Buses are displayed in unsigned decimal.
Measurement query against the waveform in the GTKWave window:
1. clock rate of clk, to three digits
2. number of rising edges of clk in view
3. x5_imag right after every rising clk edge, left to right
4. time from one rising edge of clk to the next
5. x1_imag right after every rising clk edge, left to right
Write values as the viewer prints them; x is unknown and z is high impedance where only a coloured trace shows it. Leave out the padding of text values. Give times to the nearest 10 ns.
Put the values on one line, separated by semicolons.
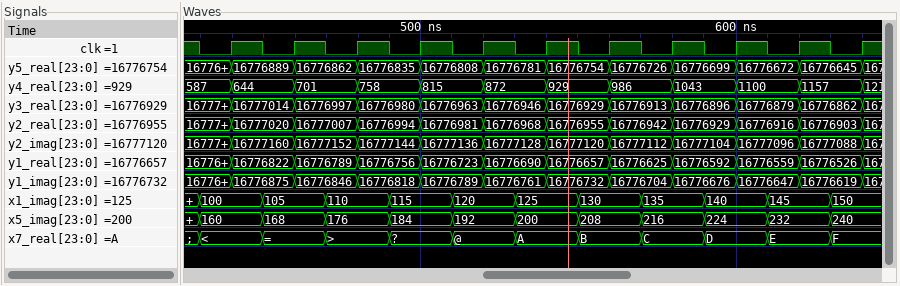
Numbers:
50.0 MHz; 11; 160, 168, 176, 184, 192, 200, 208, 216, 224, 232, 240; 20 ns; 100, 105, 110, 115, 120, 125, 130, 135, 140, 145, 150
